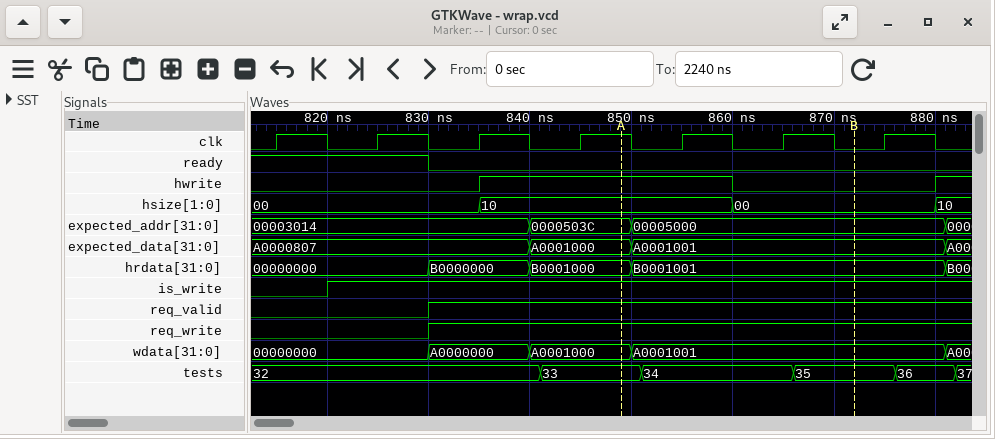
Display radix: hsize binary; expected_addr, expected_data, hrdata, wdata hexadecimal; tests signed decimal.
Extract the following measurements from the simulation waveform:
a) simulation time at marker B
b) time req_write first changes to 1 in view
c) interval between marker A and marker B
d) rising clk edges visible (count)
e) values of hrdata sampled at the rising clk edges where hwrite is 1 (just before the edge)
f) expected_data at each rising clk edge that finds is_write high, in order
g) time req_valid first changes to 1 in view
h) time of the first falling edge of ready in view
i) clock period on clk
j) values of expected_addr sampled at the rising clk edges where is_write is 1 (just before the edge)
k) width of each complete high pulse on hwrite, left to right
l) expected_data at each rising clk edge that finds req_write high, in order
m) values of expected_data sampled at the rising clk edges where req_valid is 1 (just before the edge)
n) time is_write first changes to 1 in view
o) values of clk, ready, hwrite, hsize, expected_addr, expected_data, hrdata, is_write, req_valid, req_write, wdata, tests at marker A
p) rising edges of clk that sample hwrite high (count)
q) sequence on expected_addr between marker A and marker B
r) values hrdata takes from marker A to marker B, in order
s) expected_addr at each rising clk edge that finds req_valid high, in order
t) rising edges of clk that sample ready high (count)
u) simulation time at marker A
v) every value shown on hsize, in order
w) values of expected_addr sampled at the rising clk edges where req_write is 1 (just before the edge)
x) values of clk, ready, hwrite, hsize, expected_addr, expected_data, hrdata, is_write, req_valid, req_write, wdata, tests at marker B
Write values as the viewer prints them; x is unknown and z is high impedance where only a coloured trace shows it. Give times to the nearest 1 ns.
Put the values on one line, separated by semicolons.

872 ns; 830 ns; 23 ns; 7; B0001000, B0001001; A0000807, A0000807, A0001000, A0001001, A0001001, A0001001; 830 ns; 830 ns; 10 ns; 00003014, 00003014, 0000503C, 00005000, 00005000, 00005000; 25 ns; A0000807, A0001000, A0001001, A0001001, A0001001; A0000807, A0001000, A0001001, A0001001, A0001001; 820 ns; clk=1, ready=0, hwrite=1, hsize=10, expected_addr=0000503C, expected_data=A0001000, hrdata=B0001000, is_write=1, req_valid=1, req_write=1, wdata=A0001000, tests=33; 2; 0000503C, 00005000; B0001000, B0001001; 00003014, 0000503C, 00005000, 00005000, 00005000; 2; 849 ns; 00, 10, 00, 10; 00003014, 0000503C, 00005000, 00005000, 00005000; clk=0, ready=0, hwrite=0, hsize=00, expected_addr=00005000, expected_data=A0001001, hrdata=B0001001, is_write=1, req_valid=1, req_write=1, wdata=A0001001, tests=35
